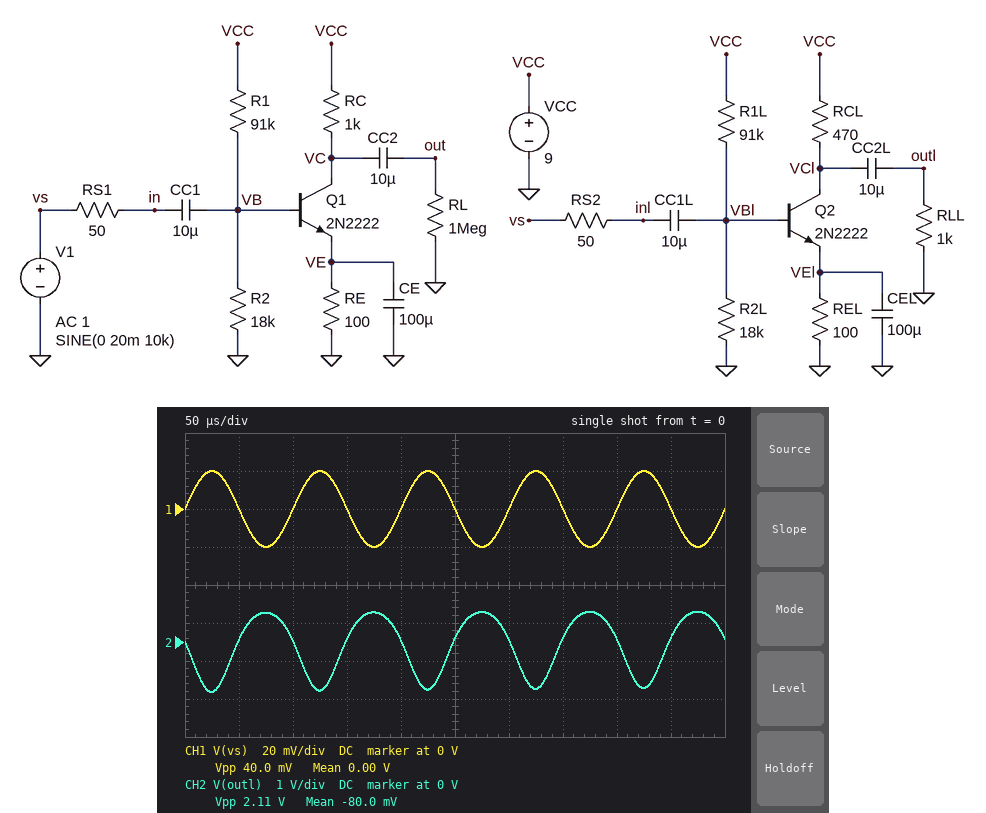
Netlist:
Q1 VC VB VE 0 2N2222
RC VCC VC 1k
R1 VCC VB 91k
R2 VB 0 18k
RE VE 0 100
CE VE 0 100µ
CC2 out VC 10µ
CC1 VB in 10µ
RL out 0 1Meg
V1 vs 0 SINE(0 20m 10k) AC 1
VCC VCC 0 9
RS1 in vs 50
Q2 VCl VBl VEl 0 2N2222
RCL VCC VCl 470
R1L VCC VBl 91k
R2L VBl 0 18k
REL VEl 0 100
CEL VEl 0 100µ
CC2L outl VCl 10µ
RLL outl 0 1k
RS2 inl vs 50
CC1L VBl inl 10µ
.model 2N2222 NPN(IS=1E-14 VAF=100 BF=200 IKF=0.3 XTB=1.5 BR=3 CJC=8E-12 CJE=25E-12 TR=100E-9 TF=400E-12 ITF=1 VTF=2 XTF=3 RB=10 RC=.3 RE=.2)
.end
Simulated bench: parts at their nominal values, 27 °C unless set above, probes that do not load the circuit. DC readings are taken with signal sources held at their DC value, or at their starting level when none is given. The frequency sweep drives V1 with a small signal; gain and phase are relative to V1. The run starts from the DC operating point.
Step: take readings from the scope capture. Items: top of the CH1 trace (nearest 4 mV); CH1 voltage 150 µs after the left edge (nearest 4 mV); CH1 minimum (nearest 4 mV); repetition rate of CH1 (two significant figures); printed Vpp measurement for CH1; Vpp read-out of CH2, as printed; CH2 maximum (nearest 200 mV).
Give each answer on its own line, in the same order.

20 mV
0 V
-20 mV
10 kHz
40.0 mV
2.11 V
800 mV
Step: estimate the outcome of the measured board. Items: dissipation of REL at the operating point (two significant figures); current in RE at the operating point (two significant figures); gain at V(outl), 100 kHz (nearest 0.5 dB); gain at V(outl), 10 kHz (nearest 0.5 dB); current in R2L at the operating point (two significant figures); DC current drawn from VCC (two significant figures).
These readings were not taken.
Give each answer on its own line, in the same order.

2.1 mW
4.6 mA
34.0 dB
34.0 dB
64 µA
9.3 mA
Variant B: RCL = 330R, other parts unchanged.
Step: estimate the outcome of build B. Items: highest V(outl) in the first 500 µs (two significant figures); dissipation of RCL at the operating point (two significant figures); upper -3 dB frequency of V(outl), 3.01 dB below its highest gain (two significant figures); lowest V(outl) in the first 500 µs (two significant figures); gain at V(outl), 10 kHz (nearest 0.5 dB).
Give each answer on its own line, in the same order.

620 mV
7.0 mW
10 MHz
-1.0 V
32.0 dB
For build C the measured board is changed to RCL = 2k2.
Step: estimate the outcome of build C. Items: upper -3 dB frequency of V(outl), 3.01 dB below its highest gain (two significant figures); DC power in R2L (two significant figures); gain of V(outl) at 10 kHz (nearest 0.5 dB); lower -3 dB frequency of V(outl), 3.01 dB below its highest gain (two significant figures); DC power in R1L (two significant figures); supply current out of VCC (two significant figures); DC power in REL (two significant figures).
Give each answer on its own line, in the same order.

860 kHz
65 µW
29.0 dB
220 Hz
690 µW
8.6 mA
1.5 mW
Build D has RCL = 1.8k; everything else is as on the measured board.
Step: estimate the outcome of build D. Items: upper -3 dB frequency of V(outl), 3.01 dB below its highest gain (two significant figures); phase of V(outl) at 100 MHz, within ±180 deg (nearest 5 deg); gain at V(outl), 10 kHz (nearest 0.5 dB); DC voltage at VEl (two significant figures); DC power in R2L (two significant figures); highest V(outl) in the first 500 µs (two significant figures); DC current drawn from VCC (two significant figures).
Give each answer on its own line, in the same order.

2.5 MHz
70 deg
40.0 dB
450 mV
73 µW
1.5 V
9.2 mA
